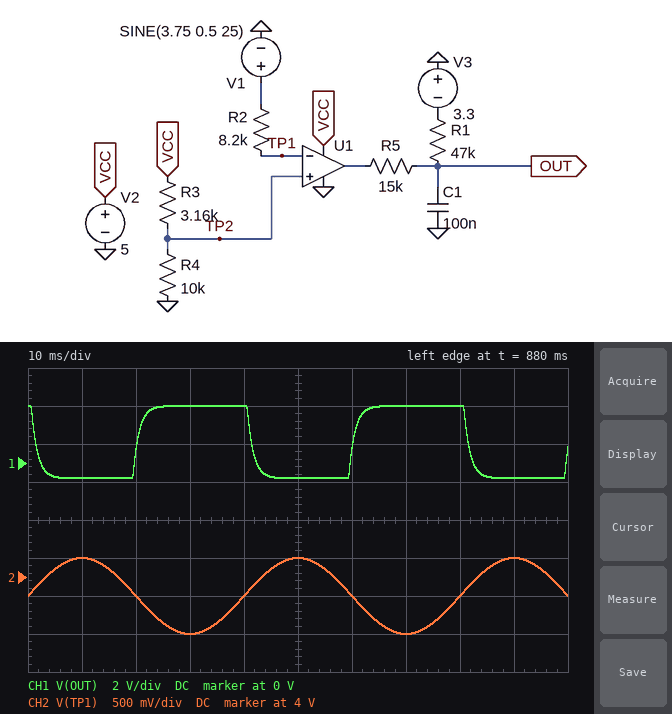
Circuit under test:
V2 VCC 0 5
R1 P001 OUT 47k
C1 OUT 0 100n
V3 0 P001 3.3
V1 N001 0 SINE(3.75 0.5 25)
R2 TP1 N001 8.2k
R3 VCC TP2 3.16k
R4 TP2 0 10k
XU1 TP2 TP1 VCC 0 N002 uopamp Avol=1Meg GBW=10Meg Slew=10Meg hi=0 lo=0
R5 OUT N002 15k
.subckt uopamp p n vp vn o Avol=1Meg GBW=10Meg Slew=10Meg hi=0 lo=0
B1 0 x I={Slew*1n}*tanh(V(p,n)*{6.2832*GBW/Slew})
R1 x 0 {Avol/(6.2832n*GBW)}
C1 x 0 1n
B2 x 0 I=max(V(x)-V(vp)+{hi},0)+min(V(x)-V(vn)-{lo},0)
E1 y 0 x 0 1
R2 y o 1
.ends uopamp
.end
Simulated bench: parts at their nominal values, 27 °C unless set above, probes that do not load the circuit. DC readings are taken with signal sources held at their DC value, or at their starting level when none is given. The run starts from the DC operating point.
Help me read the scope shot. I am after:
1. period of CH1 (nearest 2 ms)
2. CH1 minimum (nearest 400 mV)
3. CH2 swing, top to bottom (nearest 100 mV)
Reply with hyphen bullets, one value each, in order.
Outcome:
- 40 ms
- -800 mV
- 1.0 V
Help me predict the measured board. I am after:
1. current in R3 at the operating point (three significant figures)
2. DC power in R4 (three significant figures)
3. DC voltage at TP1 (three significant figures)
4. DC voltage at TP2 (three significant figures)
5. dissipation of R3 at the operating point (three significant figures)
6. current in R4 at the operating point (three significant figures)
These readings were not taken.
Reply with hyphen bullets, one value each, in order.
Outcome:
- 380 µA
- 1.44 mW
- 3.75 V
- 3.80 V
- 456 µW
- 380 µA
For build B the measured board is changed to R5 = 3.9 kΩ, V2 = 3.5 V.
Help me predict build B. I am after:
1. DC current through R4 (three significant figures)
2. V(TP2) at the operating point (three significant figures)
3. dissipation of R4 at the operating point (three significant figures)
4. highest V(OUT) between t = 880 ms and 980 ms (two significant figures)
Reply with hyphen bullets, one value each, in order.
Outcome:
- 266 µA
- 2.66 V
- 707 µW
- -260 mV
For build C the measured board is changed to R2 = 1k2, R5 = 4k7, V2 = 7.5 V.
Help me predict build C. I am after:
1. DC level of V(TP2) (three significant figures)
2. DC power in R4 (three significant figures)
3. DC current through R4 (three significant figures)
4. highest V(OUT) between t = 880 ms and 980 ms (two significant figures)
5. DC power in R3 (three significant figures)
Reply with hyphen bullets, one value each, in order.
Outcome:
- 5.70 V
- 3.25 mW
- 570 µA
- 6.5 V
- 1.03 mW
